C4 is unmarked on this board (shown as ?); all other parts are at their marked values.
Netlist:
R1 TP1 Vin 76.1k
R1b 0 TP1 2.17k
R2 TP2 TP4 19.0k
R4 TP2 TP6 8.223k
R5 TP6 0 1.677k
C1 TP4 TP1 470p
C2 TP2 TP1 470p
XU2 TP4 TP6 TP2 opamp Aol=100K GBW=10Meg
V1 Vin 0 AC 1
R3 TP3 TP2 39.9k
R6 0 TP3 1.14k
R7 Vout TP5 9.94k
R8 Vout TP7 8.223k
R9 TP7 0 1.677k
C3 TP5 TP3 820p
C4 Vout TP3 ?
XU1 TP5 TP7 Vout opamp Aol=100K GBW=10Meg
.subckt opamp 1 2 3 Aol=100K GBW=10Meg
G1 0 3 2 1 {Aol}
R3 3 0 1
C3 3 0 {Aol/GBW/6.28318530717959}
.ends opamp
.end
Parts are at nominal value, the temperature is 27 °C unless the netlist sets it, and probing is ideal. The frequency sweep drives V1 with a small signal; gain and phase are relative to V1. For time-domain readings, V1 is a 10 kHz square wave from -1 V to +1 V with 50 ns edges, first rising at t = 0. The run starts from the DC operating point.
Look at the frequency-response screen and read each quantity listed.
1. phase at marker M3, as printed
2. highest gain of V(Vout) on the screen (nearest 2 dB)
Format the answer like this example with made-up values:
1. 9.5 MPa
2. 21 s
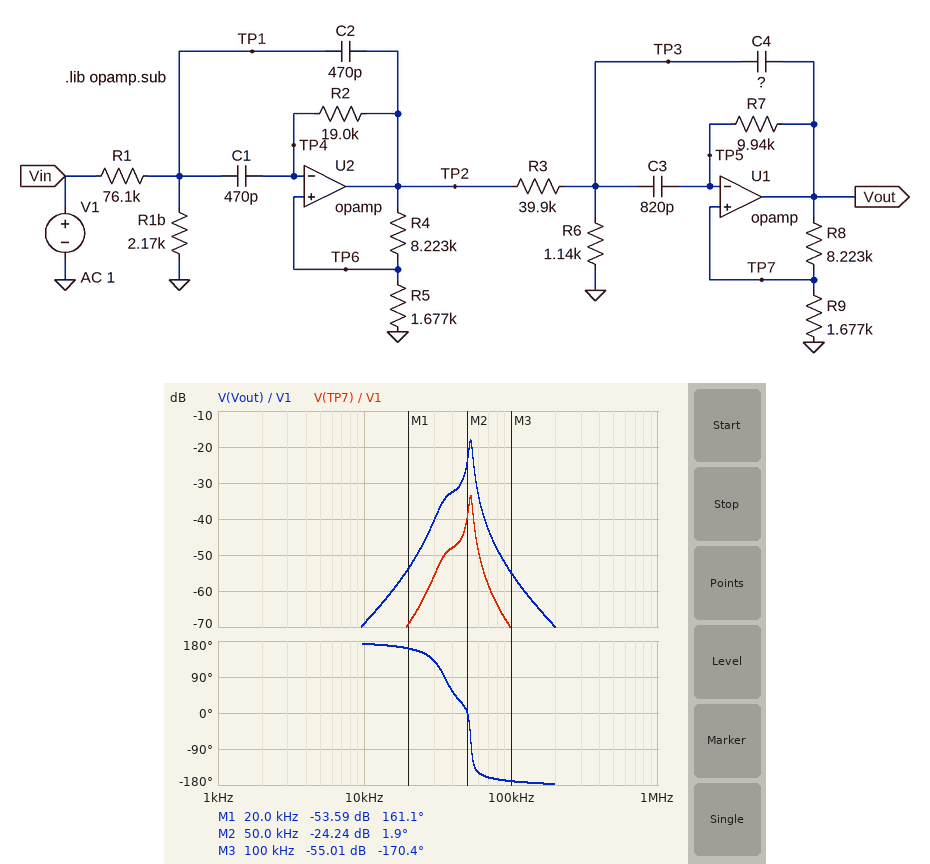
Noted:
1. -170.4 deg
2. -18 dB
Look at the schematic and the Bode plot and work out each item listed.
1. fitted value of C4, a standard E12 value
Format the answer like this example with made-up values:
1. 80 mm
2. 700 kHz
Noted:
1. 2.2 nF
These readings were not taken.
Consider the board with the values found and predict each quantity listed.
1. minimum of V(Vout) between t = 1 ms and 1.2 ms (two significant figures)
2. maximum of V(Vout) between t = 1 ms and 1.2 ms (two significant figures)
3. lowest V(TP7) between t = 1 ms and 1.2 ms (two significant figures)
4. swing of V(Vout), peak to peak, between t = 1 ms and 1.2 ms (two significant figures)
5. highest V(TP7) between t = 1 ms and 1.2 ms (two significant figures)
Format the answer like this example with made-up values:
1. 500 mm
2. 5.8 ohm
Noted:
1. -21 mV
2. 21 mV
3. -3.5 mV
4. 42 mV
5. 3.5 mV
